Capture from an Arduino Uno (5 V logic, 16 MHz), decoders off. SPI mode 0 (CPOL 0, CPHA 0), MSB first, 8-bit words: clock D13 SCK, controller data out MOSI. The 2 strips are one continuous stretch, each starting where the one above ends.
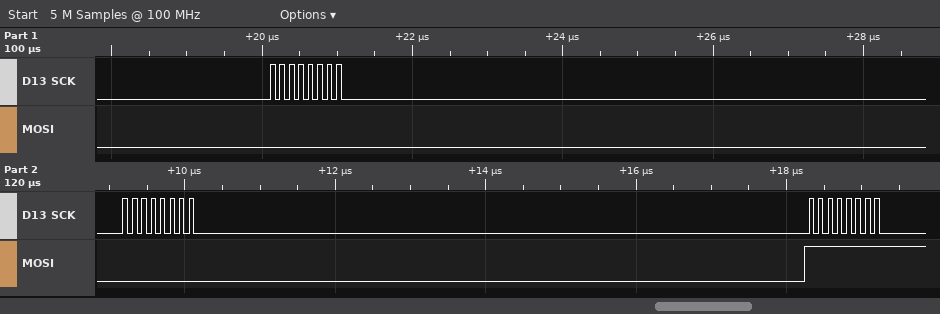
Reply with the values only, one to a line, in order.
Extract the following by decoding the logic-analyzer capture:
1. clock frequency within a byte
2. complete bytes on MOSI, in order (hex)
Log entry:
8 MHz
00 00 FF
